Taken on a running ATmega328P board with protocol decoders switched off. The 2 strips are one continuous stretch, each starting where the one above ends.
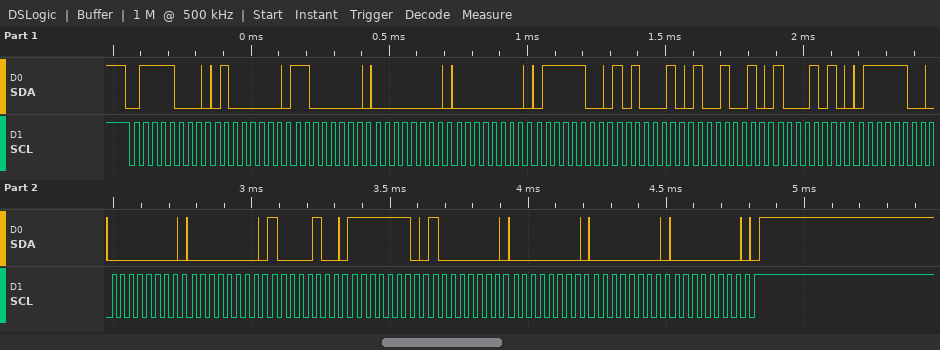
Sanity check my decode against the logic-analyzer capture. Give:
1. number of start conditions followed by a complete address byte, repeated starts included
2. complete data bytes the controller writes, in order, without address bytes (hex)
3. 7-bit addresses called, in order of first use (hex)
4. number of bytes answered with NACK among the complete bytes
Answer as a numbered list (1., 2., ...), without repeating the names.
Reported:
1. 1
2. 40 C0 00 00 7C A2 92 8A 7C 00 00 84 FE 80 00 00 00
3. 0x3C
4. 0
